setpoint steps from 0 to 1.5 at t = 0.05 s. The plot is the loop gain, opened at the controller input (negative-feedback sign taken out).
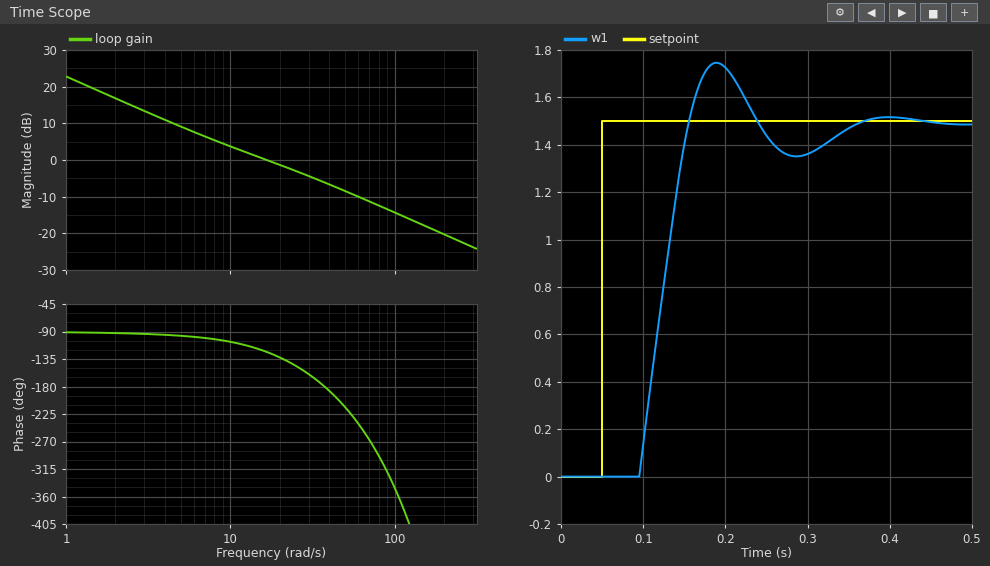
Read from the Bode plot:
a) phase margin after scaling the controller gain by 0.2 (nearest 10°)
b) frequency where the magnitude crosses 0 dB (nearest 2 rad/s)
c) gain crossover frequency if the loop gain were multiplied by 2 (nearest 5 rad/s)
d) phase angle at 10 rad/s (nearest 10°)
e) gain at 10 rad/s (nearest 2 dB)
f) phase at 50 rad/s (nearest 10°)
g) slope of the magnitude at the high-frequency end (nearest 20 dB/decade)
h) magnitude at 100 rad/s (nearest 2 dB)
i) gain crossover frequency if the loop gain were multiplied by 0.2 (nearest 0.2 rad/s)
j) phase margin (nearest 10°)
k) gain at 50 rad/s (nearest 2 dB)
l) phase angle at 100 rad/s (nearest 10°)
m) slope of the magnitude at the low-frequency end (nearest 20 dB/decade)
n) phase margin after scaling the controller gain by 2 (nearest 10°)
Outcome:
90°
16 rad/s
35 rad/s
-110°
4 dB
-210°
-20 dB/decade
-14 dB
2.8 rad/s
60°
-8 dB
-350°
-20 dB/decade
0°
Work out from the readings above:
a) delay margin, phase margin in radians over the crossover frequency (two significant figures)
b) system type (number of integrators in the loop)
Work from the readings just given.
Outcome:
0.065 s
1
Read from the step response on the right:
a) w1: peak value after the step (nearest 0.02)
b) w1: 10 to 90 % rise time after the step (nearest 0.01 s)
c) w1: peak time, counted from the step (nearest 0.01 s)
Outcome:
1.74
0.05 s
0.14 s
